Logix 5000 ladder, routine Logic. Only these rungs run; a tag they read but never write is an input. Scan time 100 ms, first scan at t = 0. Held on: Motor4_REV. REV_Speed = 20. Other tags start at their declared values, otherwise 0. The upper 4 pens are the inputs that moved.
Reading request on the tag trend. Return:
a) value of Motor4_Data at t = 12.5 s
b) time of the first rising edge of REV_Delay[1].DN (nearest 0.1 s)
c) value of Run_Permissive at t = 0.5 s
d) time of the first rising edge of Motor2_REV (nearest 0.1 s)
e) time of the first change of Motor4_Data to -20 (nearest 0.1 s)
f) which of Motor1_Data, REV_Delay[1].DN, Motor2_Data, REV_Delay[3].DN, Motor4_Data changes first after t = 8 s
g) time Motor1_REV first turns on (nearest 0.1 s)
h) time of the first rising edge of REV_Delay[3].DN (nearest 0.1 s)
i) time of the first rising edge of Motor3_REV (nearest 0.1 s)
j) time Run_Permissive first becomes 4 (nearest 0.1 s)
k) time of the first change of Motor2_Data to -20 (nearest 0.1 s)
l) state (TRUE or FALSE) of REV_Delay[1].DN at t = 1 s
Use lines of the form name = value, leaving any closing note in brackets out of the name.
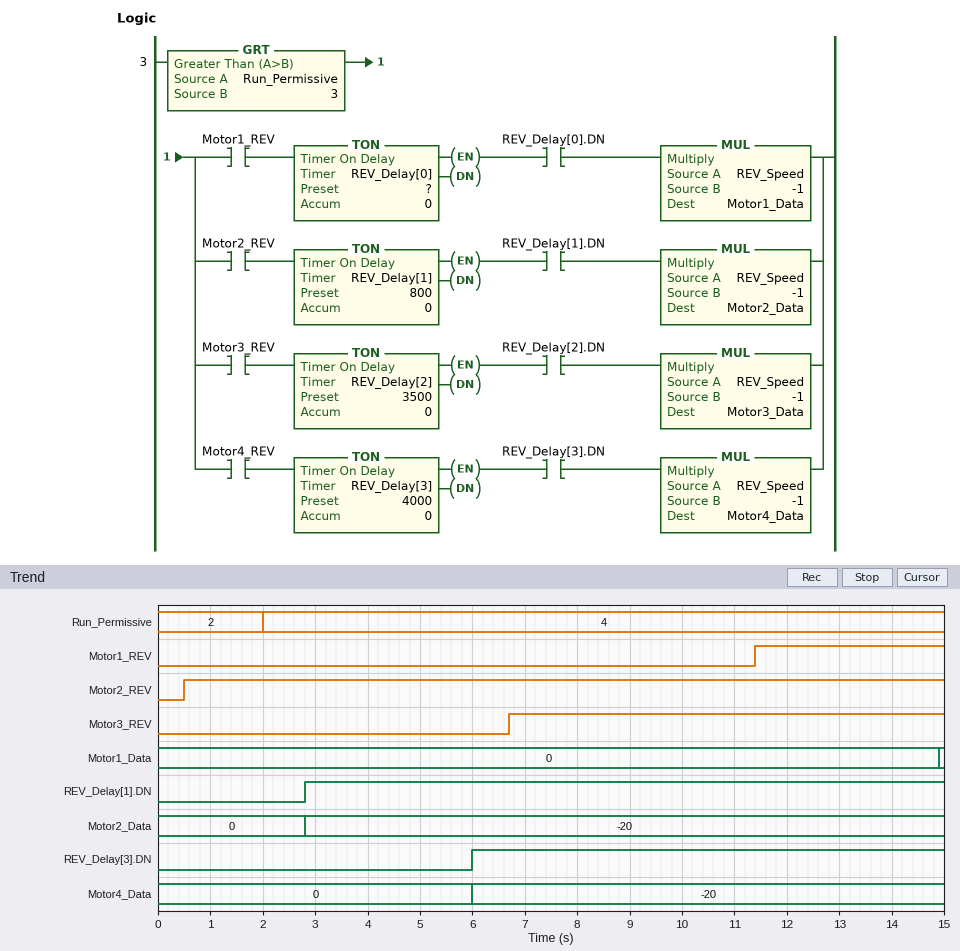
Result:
value of Motor4_Data at t = 12.5 s = -20
time of the first rising edge of REV_Delay[1].DN = 2.8 s
value of Run_Permissive at t = 0.5 s = 2
time of the first rising edge of Motor2_REV = 0.5 s
time of the first change of Motor4_Data to -20 = 6.0 s
which of Motor1_Data, REV_Delay[1].DN, Motor2_Data, REV_Delay[3].DN, Motor4_Data changes first after t = 8 s = Motor1_Data
time Motor1_REV first turns on = 11.4 s
time of the first rising edge of REV_Delay[3].DN = 6.0 s
time of the first rising edge of Motor3_REV = 6.7 s
time Run_Permissive first becomes 4 = 2.0 s
time of the first change of Motor2_Data to -20 = 2.8 s
state (TRUE or FALSE) of REV_Delay[1].DN at t = 1 s = FALSE
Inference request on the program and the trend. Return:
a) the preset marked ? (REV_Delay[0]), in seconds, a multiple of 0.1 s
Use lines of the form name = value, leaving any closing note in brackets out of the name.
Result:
the preset marked ? (REV_Delay[0]), in seconds, a multiple of 0.1 s = 3.5 s
